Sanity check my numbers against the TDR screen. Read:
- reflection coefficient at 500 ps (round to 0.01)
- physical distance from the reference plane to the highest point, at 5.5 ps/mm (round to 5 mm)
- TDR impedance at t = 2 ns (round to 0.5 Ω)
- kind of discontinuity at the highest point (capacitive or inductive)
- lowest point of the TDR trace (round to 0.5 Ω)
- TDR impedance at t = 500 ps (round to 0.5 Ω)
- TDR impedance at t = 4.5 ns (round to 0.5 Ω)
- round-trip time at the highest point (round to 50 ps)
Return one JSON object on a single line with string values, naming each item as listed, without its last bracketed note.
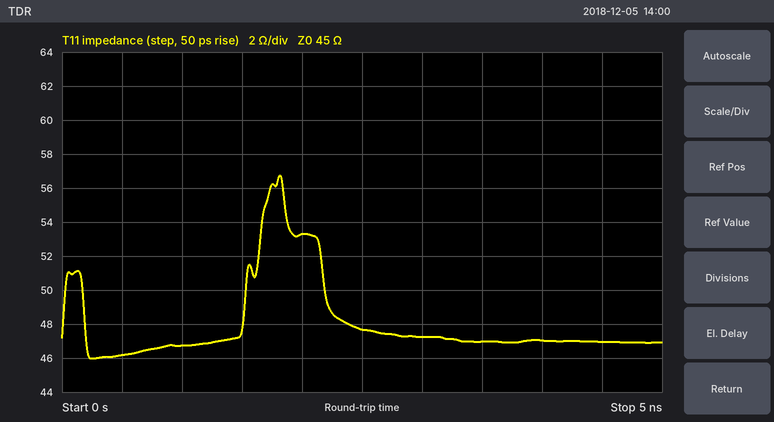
{"reflection coefficient at 500 ps": "+0.01", "physical distance from the reference plane to the highest point, at 5.5 ps/mm": "165 mm", "TDR impedance at t = 2 ns": "53.5 Ω", "kind of discontinuity at the highest point": "inductive", "lowest point of the TDR trace": "46.0 Ω", "TDR impedance at t = 500 ps": "46.0 Ω", "TDR impedance at t = 4.5 ns": "47.0 Ω", "round-trip time at the highest point": "1.80 ns"}
